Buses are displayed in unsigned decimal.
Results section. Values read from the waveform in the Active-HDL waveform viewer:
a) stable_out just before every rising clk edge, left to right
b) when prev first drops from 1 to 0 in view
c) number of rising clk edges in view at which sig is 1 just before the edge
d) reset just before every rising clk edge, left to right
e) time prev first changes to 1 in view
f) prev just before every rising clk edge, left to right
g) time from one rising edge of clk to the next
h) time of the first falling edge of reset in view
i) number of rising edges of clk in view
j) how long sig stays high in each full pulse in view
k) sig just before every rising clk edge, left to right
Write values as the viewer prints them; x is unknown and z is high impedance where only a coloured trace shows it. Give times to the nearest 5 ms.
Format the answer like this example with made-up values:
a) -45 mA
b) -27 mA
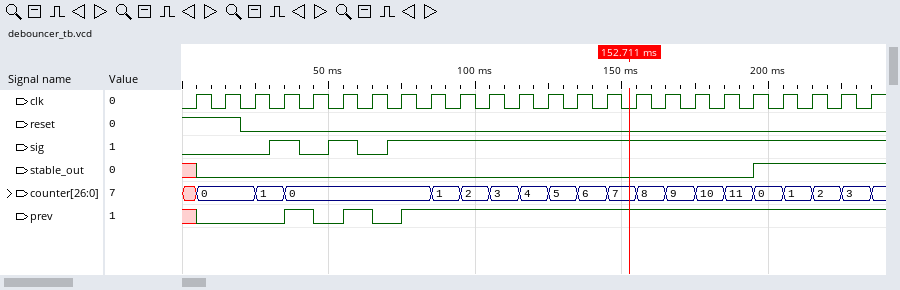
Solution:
a) x 0 0 0 0 0 0 0 0 0 0 0 0 0 0 0 0 0 0 0 1 1 1 1
b) 45 ms
c) 19
d) 1 1 0 0 0 0 0 0 0 0 0 0 0 0 0 0 0 0 0 0 0 0 0 0
e) 35 ms
f) x 0 0 0 1 0 1 0 1 1 1 1 1 1 1 1 1 1 1 1 1 1 1 1
g) 10 ms
h) 20 ms
i) 24
j) 10 ms, 10 ms
k) 0 0 0 1 0 1 0 1 1 1 1 1 1 1 1 1 1 1 1 1 1 1 1 1
